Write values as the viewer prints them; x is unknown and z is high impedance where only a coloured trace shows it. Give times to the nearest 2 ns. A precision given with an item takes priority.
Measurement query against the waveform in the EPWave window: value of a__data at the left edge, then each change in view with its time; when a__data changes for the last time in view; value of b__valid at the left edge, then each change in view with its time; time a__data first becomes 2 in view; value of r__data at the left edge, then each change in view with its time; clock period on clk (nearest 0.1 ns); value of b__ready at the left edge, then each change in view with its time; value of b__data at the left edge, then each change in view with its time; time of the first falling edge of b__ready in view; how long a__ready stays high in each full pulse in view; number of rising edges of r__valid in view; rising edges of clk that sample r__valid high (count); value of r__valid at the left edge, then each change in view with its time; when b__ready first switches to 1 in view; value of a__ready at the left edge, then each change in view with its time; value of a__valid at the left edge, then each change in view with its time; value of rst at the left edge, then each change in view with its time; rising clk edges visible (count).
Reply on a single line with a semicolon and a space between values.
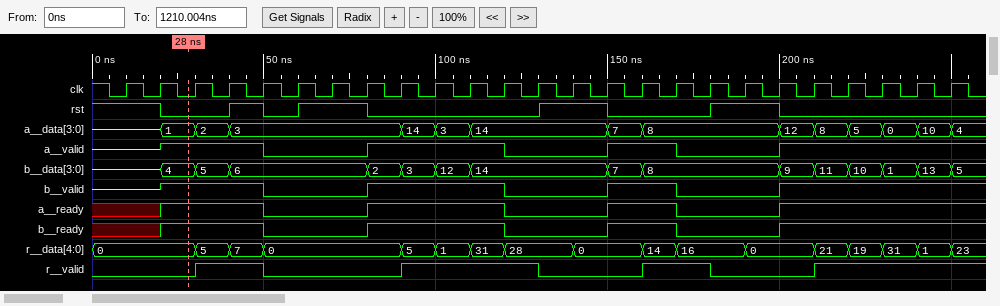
z, 1 at 20 ns, 2 at 30 ns, 3 at 40 ns, 14 at 90 ns, 3 at 100 ns, 14 at 110 ns, 7 at 150 ns, 8 at 160 ns, 12 at 200 ns, 8 at 210 ns, 5 at 220 ns, 0 at 230 ns, 10 at 240 ns, 4 at 250 ns; 250 ns; z, 1 at 20 ns, 0 at 50 ns, 1 at 80 ns, 0 at 120 ns, 1 at 150 ns, 0 at 170 ns, 1 at 200 ns; 30 ns; 0, 5 at 30 ns, 7 at 40 ns, 0 at 50 ns, 5 at 90 ns, 1 at 100 ns, 31 at 110 ns, 28 at 120 ns, 0 at 140 ns, 14 at 160 ns, 16 at 170 ns, 0 at 190 ns, 21 at 210 ns, 19 at 220 ns, 31 at 230 ns, 1 at 240 ns, 23 at 250 ns; 10 ns; x, 1 at 20 ns, 0 at 50 ns, 1 at 80 ns, 0 at 120 ns, 1 at 150 ns, 0 at 170 ns, 1 at 200 ns; z, 4 at 20 ns, 5 at 30 ns, 6 at 40 ns, 2 at 80 ns, 3 at 90 ns, 12 at 100 ns, 14 at 110 ns, 7 at 150 ns, 8 at 160 ns, 9 at 200 ns, 11 at 210 ns, 10 at 220 ns, 1 at 230 ns, 13 at 240 ns, 5 at 250 ns; 50 ns; 40 ns, 20 ns; 4; 12; 0, 1 at 30 ns, 0 at 50 ns, 1 at 90 ns, 0 at 130 ns, 1 at 160 ns, 0 at 180 ns, 1 at 210 ns; 20 ns; x, 1 at 20 ns, 0 at 50 ns, 1 at 80 ns, 0 at 120 ns, 1 at 150 ns, 0 at 170 ns, 1 at 200 ns; z, 1 at 20 ns, 0 at 50 ns, 1 at 80 ns, 0 at 120 ns, 1 at 150 ns, 0 at 170 ns, 1 at 200 ns; 1, 0 at 20 ns, 1 at 40 ns, 0 at 50 ns, 1 at 60 ns, 0 at 80 ns, 1 at 130 ns, 0 at 150 ns, 1 at 180 ns, 0 at 200 ns; 25
